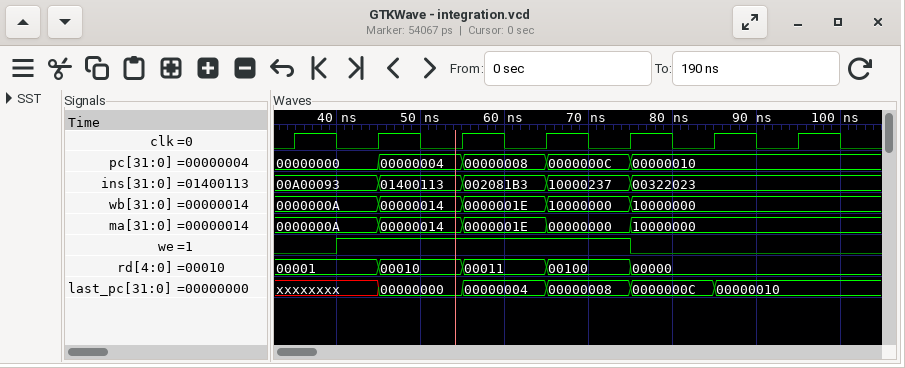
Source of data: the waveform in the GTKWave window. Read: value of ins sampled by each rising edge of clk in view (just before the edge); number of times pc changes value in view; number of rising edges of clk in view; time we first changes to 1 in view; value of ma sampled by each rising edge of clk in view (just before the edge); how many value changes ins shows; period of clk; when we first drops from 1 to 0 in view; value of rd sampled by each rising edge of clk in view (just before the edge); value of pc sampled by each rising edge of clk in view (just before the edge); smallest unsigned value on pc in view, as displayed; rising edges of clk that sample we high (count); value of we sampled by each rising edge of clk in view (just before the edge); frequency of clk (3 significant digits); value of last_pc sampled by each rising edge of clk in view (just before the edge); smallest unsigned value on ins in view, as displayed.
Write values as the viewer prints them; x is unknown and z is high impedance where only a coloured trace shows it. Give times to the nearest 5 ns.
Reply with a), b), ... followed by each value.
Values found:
a) 00A00093, 00A00093, 01400113, 002081B3, 10000237, 00322023, 00322023
b) 4
c) 7
d) 40 ns
e) 0000000A, 0000000A, 00000014, 0000001E, 00000000, 10000000, 10000000
f) 4
g) 10 ns
h) 75 ns
i) 00001, 00001, 00010, 00011, 00100, 00000, 00000
j) 00000000, 00000000, 00000004, 00000008, 0000000C, 00000010, 00000010
k) 00000000
l) 4
m) 0 1 1 1 1 0 0
n) 100 MHz
o) xxxxxxxx, xxxxxxxx, 00000000, 00000004, 00000008, 0000000C, 00000010
p) 002081B3
